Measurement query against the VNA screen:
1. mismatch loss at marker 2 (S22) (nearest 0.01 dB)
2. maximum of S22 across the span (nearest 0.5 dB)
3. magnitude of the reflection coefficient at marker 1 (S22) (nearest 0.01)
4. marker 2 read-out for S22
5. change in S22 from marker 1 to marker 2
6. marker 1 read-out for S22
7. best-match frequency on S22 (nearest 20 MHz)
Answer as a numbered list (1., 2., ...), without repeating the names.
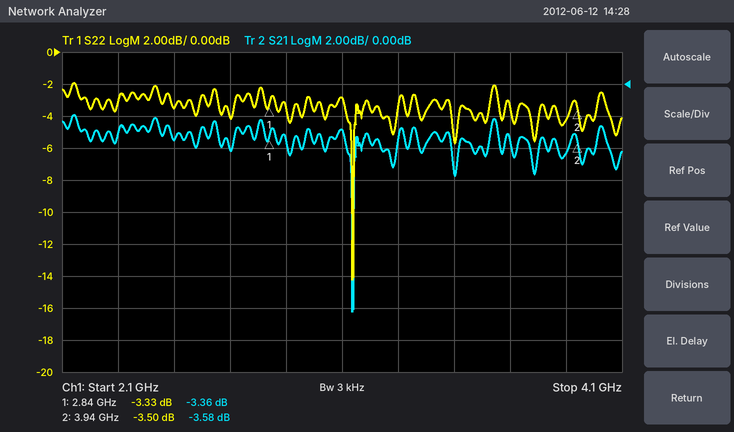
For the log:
1. 2.57 dB
2. -2.0 dB
3. 0.68
4. -3.50 dB
5. -0.17 dB
6. -3.33 dB
7. 3.14 GHz
